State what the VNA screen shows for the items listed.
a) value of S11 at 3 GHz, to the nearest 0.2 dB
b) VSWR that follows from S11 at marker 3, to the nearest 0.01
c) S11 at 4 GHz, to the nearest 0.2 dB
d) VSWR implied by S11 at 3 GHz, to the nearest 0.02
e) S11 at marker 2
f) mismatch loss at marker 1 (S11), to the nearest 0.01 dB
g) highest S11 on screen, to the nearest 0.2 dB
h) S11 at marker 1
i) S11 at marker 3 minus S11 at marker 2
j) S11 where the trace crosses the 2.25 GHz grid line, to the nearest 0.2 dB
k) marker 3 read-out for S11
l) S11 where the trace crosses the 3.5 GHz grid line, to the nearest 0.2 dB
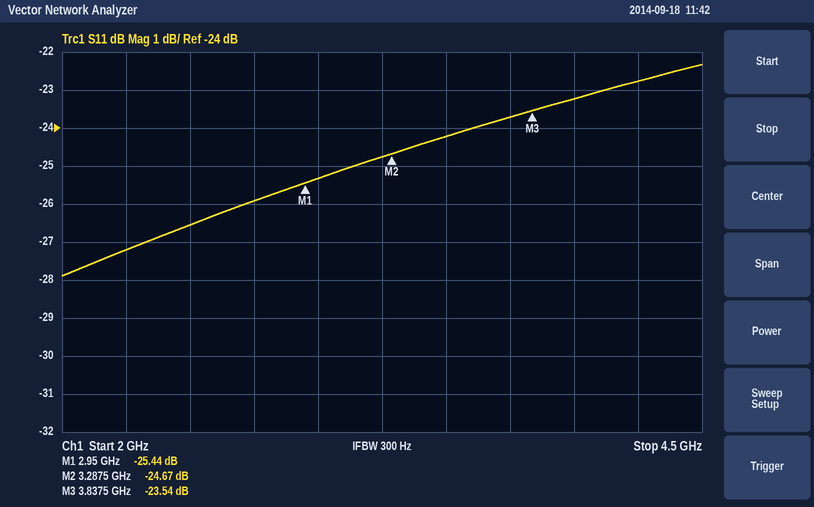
-25.4 dB
1.14
-23.2 dB
1.12
-24.67 dB
0.01 dB
-22.4 dB
-25.44 dB
1.13 dB
-27.2 dB
-23.54 dB
-24.2 dB
